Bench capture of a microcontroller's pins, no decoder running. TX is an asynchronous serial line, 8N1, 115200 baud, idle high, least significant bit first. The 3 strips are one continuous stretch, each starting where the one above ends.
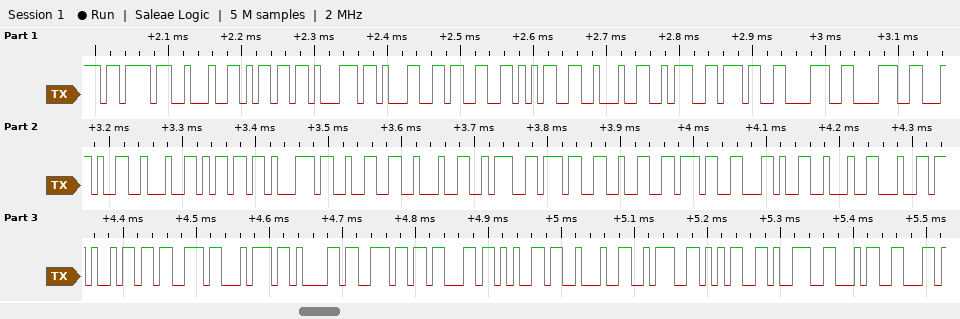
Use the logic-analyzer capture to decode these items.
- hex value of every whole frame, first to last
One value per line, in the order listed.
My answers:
0x7B 0x22 0x6D 0x71 0x31 0x33 0x35 0x22 0x3A 0x37 0x38 0x38 0x2C 0x22 0x6D 0x71 0x32 0x22 0x3A 0x37 0x32 0x37 0x2C 0x22 0x64 0x69 0x73 0x74 0x61 0x6E 0x63 0x65 0x22 0x3A 0x35 0x39 0x34
